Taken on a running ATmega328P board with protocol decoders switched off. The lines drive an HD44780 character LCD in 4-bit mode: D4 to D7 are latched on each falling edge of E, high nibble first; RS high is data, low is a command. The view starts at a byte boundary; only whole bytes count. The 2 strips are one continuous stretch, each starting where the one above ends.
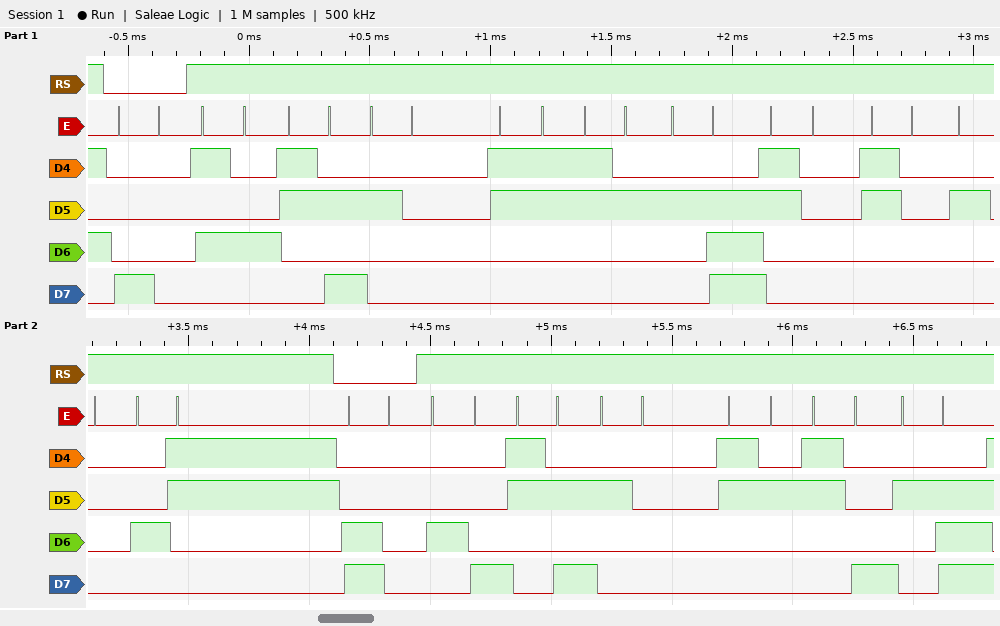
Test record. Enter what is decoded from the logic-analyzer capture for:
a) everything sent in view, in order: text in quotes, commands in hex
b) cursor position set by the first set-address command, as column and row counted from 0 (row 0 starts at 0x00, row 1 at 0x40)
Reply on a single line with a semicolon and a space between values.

0x80 "T: 32.00 C" 0xC0 "H: 28."; column 0, row 0
